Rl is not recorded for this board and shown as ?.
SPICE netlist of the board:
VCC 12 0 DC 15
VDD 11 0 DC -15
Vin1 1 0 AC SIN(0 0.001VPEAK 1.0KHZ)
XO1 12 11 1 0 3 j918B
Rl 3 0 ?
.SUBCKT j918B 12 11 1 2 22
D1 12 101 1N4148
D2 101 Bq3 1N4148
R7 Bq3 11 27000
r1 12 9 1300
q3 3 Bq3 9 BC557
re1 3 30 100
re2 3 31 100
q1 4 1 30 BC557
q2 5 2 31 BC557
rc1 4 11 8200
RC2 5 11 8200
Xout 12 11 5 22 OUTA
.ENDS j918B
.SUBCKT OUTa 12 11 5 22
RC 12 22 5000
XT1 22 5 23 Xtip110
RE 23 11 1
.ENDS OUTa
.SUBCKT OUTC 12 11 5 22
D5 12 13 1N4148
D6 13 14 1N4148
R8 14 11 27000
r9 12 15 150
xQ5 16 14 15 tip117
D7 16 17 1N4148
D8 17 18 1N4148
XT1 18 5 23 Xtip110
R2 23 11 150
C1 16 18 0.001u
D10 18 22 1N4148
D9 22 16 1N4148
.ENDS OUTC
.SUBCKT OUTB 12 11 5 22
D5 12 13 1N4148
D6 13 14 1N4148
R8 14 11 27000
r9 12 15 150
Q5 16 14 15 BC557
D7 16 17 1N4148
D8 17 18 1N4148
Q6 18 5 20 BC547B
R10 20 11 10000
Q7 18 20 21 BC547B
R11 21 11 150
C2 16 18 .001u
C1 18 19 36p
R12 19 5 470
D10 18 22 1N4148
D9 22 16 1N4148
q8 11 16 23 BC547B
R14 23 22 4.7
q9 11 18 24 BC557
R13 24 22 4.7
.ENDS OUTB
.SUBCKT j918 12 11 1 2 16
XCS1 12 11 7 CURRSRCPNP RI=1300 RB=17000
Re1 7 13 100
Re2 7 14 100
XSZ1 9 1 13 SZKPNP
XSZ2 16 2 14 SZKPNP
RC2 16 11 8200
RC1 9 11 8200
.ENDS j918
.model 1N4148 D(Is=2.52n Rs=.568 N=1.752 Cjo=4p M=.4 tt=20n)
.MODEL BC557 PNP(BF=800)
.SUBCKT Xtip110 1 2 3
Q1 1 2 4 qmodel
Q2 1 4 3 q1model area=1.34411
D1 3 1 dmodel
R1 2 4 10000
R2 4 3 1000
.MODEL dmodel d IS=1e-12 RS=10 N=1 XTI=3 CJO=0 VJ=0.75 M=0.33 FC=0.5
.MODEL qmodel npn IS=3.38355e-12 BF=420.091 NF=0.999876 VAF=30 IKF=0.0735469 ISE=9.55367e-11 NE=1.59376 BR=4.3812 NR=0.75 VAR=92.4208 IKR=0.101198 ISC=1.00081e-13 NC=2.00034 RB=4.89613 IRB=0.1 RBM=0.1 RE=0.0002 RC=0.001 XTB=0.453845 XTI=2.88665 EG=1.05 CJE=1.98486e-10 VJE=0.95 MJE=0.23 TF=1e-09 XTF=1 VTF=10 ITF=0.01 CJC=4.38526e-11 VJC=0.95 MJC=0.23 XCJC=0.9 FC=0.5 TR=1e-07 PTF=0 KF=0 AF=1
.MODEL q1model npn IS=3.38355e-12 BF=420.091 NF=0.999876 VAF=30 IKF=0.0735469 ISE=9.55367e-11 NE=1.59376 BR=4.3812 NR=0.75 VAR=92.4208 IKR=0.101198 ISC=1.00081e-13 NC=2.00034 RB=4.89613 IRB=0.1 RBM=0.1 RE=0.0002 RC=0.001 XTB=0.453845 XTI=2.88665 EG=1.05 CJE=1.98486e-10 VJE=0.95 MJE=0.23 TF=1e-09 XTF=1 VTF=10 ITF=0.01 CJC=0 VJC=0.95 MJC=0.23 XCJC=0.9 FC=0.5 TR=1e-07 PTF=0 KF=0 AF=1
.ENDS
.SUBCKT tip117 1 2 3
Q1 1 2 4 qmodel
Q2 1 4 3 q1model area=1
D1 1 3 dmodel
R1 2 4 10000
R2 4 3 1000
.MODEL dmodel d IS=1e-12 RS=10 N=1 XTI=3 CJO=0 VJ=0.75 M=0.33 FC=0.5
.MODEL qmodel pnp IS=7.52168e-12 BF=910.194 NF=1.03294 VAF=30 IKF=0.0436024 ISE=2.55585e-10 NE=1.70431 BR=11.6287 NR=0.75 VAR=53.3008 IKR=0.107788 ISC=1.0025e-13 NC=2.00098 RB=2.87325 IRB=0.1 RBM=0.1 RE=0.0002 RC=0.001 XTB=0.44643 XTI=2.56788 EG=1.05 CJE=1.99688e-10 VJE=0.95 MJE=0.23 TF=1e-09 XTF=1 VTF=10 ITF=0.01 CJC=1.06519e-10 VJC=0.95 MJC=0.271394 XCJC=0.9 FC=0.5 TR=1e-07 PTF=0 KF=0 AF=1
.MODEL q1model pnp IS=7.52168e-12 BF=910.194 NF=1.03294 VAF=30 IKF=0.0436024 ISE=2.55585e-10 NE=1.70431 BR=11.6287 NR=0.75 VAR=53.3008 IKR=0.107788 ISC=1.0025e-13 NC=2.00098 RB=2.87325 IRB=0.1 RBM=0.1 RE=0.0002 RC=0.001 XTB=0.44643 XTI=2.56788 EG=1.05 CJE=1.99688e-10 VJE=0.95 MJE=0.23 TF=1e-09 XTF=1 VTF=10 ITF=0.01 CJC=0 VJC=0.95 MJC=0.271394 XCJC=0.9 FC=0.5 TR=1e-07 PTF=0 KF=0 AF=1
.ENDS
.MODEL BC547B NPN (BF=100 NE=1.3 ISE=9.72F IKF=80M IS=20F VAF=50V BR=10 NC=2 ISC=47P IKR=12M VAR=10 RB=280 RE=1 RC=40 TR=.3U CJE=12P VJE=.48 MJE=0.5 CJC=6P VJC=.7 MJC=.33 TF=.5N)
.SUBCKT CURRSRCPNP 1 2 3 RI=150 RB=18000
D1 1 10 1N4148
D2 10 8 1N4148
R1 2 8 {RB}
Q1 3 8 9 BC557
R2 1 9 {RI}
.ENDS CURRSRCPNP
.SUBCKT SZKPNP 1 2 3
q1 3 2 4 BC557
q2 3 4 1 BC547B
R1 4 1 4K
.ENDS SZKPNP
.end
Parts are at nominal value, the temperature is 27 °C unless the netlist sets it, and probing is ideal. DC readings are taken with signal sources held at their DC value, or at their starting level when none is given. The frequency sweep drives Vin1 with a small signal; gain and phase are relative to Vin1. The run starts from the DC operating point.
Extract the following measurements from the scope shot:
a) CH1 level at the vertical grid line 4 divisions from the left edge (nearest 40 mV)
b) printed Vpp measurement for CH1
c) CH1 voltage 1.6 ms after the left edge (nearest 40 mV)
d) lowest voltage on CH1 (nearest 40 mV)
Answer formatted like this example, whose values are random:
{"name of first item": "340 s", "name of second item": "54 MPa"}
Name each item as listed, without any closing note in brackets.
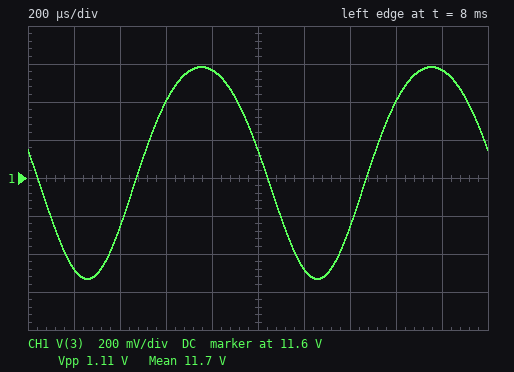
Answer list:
{"CH1 level at the vertical grid line 4 divisions from the left edge": "12.16 V", "printed Vpp measurement for CH1": "1.11 V", "CH1 voltage 1.6 ms after the left edge": "12.00 V", "lowest voltage on CH1": "11.08 V"}
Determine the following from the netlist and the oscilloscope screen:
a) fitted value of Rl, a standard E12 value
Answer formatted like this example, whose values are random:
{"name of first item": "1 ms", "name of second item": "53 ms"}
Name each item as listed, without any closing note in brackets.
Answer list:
{"fitted value of Rl, a standard E12 value": "270 kΩ"}
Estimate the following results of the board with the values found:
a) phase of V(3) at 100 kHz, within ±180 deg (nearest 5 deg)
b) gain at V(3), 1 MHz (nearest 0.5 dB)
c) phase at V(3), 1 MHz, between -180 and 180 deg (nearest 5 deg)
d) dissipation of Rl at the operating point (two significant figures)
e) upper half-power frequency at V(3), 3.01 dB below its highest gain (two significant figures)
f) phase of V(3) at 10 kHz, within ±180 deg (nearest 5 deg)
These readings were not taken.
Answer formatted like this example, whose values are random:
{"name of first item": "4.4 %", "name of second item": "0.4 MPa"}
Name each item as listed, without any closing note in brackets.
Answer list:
{"phase of V(3) at 100 kHz, within ±180 deg": "105 deg", "gain at V(3), 1 MHz": "23.0 dB", "phase at V(3), 1 MHz, between -180 and 180 deg": "90 deg", "dissipation of Rl at the operating point": "510 µW", "upper half-power frequency at V(3), 3.01 dB below its highest gain": "26 kHz", "phase of V(3) at 10 kHz, within ±180 deg": "160 deg"}
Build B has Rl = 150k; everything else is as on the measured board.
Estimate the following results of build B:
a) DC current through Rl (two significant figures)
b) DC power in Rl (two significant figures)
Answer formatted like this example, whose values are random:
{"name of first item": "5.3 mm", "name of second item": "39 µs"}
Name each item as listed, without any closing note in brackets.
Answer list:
{"DC current through Rl": "77 µA", "DC power in Rl": "890 µW"}
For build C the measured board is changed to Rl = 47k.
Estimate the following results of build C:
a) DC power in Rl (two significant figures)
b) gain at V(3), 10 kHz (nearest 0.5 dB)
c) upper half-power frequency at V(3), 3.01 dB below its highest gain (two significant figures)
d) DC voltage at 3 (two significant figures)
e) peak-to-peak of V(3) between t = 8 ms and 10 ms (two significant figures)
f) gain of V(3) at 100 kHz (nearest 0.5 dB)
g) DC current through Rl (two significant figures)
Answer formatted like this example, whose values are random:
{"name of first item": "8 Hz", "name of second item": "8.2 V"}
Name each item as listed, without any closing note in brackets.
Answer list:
{"DC power in Rl": "2.5 mW", "gain at V(3), 10 kHz": "53.0 dB", "upper half-power frequency at V(3), 3.01 dB below its highest gain": "29 kHz", "DC voltage at 3": "11 V", "peak-to-peak of V(3) between t = 8 ms and 10 ms": "980 mV", "gain of V(3) at 100 kHz": "42.5 dB", "DC current through Rl": "230 µA"}
